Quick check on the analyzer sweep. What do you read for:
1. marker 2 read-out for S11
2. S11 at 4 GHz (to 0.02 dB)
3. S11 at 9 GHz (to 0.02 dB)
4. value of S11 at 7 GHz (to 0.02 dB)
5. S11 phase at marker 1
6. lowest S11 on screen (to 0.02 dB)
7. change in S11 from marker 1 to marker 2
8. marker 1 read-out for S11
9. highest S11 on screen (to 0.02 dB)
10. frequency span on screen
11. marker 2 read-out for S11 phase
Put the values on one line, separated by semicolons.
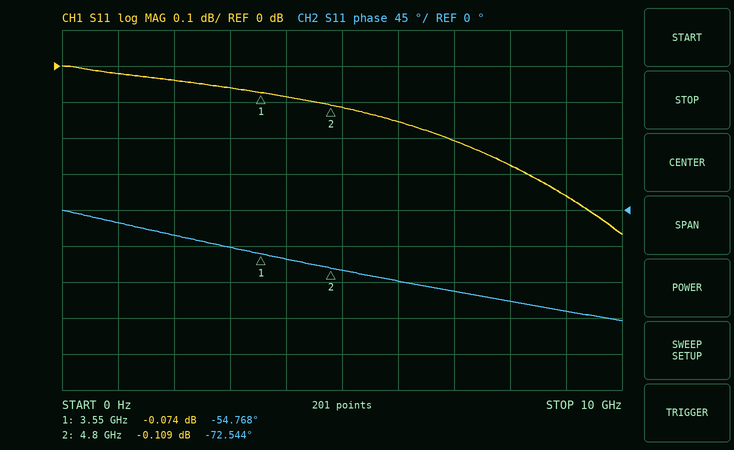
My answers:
-0.109 dB; -0.08 dB; -0.36 dB; -0.20 dB; -54.768°; -0.46 dB; -0.035 dB; -0.074 dB; 0.00 dB; 10 GHz; -72.544°
